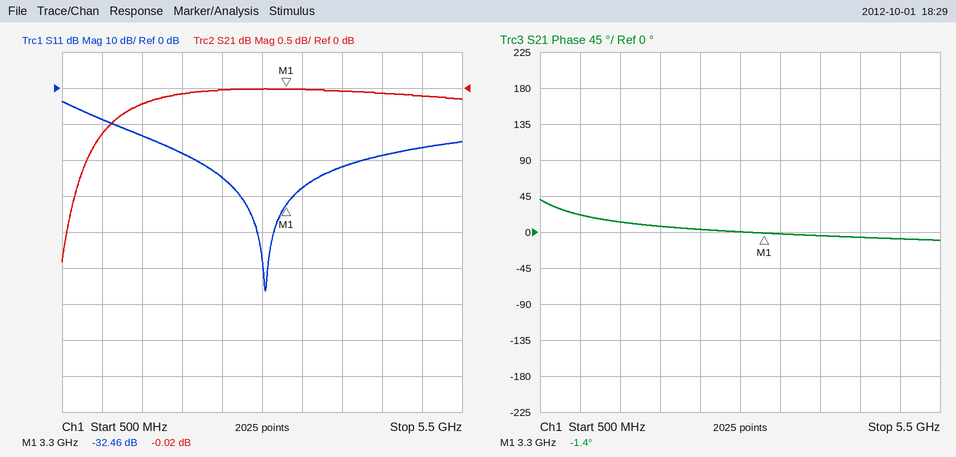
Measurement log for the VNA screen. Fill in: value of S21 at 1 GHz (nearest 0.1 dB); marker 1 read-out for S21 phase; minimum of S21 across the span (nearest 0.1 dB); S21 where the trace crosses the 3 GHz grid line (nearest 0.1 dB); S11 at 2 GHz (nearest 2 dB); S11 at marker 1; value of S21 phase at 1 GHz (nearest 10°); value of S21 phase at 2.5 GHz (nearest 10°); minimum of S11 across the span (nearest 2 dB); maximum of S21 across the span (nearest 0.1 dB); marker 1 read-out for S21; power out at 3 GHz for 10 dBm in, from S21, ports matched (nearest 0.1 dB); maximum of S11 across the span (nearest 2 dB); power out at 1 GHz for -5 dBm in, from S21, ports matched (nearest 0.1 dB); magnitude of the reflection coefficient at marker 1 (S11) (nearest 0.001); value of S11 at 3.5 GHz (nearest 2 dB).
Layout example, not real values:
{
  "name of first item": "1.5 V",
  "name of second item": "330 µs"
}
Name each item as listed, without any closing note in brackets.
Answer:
{
  "value of S21 at 1 GHz": "-0.6 dB",
  "marker 1 read-out for S21 phase": "-1.4°",
  "minimum of S21 across the span": "-2.4 dB",
  "S21 where the trace crosses the 3 GHz grid line": "0.0 dB",
  "S11 at 2 GHz": "-18 dB",
  "S11 at marker 1": "-32.46 dB",
  "value of S21 phase at 1 GHz": "20°",
  "value of S21 phase at 2.5 GHz": "0°",
  "minimum of S11 across the span": "-56 dB",
  "maximum of S21 across the span": "0.0 dB",
  "marker 1 read-out for S21": "-0.02 dB",
  "power out at 3 GHz for 10 dBm in, from S21, ports matched": "10.0 dBm",
  "maximum of S11 across the span": "-4 dB",
  "power out at 1 GHz for -5 dBm in, from S21, ports matched": "-5.6 dBm",
  "magnitude of the reflection coefficient at marker 1 (S11)": "0.024",
  "value of S11 at 3.5 GHz": "-28 dB"
}
